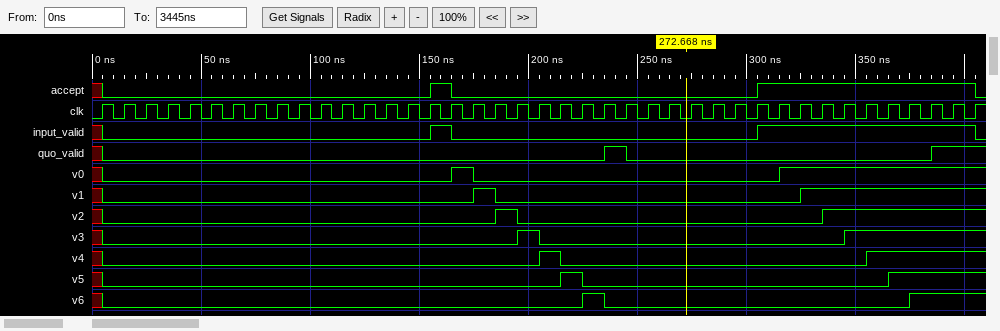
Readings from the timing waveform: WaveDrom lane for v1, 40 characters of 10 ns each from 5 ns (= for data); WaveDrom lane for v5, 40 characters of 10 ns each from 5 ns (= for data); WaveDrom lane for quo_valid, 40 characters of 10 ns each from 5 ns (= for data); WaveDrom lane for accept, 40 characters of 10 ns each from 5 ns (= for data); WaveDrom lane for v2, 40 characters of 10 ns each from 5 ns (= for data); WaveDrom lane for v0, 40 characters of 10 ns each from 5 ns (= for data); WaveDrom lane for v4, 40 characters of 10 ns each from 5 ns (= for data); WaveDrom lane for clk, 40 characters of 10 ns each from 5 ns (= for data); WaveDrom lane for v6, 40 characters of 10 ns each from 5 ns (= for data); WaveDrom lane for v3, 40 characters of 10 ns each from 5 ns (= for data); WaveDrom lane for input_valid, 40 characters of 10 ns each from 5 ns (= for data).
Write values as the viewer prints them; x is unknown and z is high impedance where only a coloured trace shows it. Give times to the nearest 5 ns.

{name: 'v1', wave: '0................10.............1.......'}
{name: 'v5', wave: '0....................10.............1...'}
{name: 'quo_valid', wave: '0......................10.............1.'}
{name: 'accept', wave: '0..............10.............1.........'}
{name: 'v2', wave: '0.................10.............1......'}
{name: 'v0', wave: '0...............10.............1........'}
{name: 'v4', wave: '0...................10.............1....'}
{name: 'clk', wave: 'p.......................................'}
{name: 'v6', wave: '0.....................10.............1..'}
{name: 'v3', wave: '0..................10.............1.....'}
{name: 'input_valid', wave: '0..............10.............1.........'}
